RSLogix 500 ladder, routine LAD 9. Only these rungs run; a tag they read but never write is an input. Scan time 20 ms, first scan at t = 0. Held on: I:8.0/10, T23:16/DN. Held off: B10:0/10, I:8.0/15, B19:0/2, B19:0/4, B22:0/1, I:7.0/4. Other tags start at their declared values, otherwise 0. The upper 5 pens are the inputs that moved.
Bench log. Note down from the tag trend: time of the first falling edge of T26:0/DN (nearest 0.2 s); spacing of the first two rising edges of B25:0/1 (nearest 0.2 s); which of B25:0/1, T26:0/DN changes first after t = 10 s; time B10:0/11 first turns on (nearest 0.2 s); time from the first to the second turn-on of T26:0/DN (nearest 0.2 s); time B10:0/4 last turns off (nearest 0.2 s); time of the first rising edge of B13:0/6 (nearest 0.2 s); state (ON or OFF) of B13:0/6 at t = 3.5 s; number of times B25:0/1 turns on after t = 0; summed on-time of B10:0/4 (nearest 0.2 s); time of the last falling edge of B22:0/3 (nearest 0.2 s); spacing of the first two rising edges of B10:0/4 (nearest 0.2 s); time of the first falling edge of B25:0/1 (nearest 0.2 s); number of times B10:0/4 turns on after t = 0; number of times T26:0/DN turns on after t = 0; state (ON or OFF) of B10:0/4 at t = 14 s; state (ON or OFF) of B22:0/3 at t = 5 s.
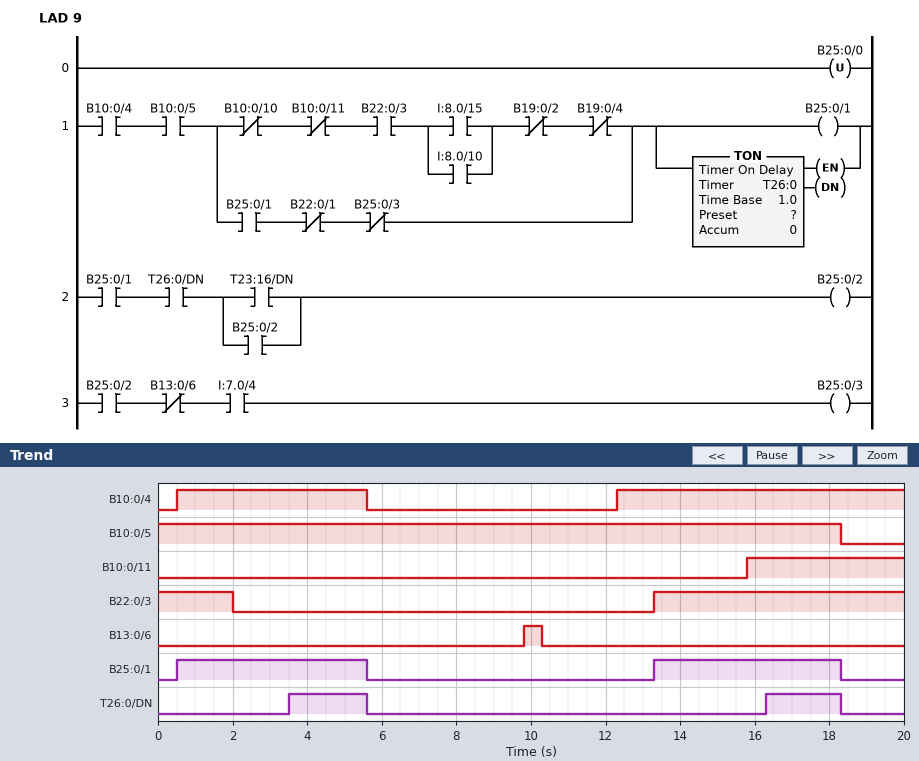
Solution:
5.6 s
12.8 s
B25:0/1
15.8 s
12.8 s
5.6 s
9.8 s
OFF
2
12.8 s
2.0 s
11.8 s
5.6 s
2
2
ON
OFF
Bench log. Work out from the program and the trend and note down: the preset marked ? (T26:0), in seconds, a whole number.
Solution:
3 s
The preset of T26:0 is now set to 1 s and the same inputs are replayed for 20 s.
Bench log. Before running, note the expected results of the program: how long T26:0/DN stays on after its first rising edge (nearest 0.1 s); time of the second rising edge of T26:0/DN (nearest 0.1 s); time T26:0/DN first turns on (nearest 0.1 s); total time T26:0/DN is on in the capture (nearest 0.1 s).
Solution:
4.1 s
14.3 s
1.5 s
8.1 s
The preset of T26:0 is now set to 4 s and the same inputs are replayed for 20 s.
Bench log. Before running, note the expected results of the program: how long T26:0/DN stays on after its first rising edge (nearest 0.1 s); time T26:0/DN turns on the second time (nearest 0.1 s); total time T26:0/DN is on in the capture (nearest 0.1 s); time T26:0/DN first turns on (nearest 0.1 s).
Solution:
1.1 s
17.3 s
2.1 s
4.5 s
